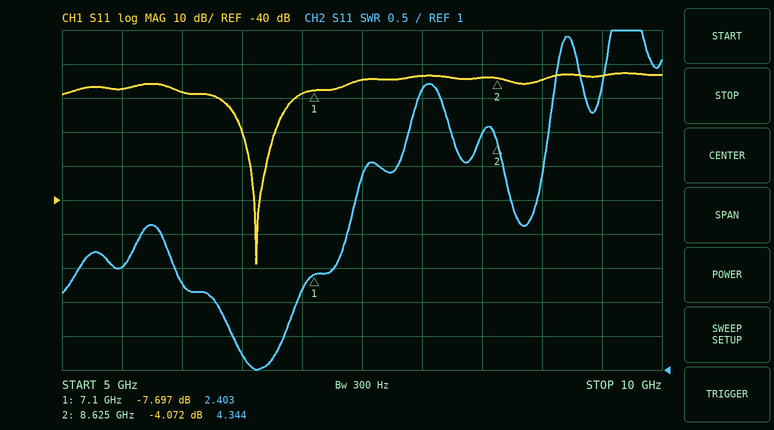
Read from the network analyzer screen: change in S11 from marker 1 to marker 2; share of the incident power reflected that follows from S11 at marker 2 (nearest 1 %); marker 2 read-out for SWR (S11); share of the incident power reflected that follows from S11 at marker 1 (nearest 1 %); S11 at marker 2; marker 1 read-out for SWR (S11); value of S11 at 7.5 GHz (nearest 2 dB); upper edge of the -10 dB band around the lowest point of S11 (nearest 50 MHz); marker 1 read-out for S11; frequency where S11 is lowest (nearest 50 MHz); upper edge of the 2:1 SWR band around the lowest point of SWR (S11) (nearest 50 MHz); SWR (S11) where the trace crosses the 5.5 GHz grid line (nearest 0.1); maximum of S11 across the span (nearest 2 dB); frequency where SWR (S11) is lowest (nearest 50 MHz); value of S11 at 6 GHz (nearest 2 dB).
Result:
3.625 dB
39 %
4.344
17 %
-4.072 dB
2.403
-4 dB
6.95 GHz
-7.697 dB
6.60 GHz
6.95 GHz
2.5
-2 dB
6.60 GHz
-8 dB
